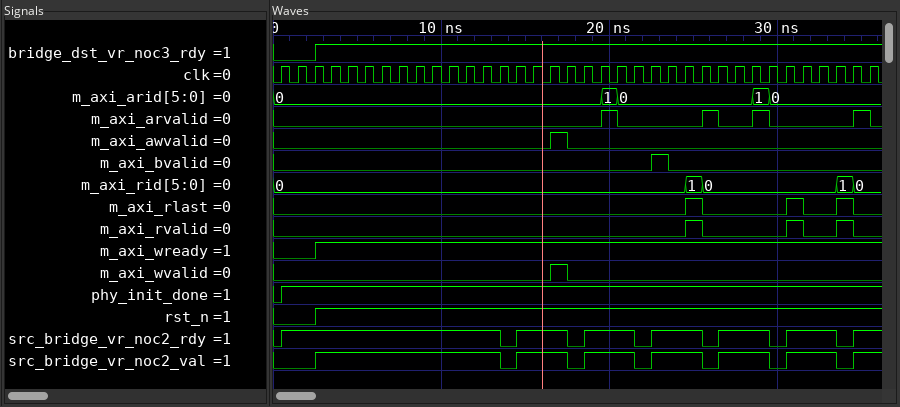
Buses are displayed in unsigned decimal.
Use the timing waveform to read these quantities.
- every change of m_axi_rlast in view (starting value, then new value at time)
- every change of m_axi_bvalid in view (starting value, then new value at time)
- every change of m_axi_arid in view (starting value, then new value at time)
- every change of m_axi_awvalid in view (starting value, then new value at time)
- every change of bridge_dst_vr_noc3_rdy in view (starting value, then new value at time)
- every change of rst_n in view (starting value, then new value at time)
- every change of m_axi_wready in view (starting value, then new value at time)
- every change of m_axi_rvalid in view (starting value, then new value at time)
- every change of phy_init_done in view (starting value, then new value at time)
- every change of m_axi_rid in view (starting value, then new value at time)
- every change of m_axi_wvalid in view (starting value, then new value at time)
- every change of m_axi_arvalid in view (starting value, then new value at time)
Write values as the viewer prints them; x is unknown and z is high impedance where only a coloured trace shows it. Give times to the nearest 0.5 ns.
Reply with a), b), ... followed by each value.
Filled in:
a) 0, 1 at 24.5 ns, 0 at 25.5 ns, 1 at 30.5 ns, 0 at 31.5 ns, 1 at 33.5 ns, 0 at 34.5 ns
b) 0, 1 at 22.5 ns, 0 at 23.5 ns
c) 0, 1 at 19.5 ns, 0 at 20.5 ns, 1 at 28.5 ns, 0 at 29.5 ns
d) 0, 1 at 16.5 ns, 0 at 17.5 ns
e) 0, 1 at 2.5 ns
f) 0, 1 at 2.5 ns
g) 0, 1 at 2.5 ns
h) 0, 1 at 24.5 ns, 0 at 25.5 ns, 1 at 30.5 ns, 0 at 31.5 ns, 1 at 33.5 ns, 0 at 34.5 ns
i) 0, 1 at 0.5 ns
j) 0, 1 at 24.5 ns, 0 at 25.5 ns, 1 at 33.5 ns, 0 at 34.5 ns
k) 0, 1 at 16.5 ns, 0 at 17.5 ns
l) 0, 1 at 19.5 ns, 0 at 20.5 ns, 1 at 25.5 ns, 0 at 26.5 ns, 1 at 28.5 ns, 0 at 29.5 ns, 1 at 34.5 ns, 0 at 35.5 ns
